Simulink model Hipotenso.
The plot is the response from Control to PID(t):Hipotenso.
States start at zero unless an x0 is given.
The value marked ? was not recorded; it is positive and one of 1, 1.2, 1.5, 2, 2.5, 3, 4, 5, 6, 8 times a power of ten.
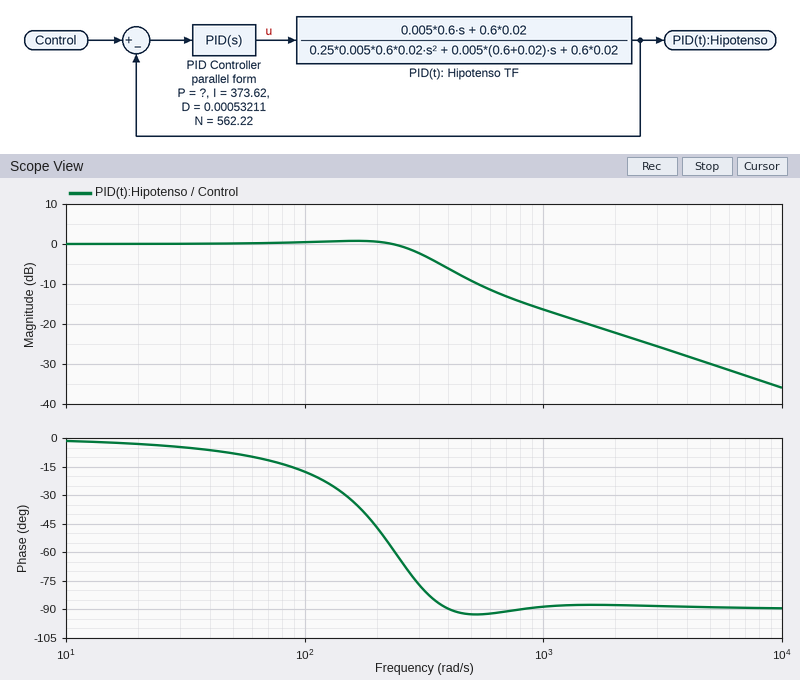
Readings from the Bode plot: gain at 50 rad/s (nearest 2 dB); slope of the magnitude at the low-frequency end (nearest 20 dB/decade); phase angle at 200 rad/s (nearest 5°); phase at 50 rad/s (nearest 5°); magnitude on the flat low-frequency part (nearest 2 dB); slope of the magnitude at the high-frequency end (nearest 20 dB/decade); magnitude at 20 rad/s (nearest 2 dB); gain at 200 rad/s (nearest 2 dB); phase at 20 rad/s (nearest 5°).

0 dB
0 dB/decade
-45°
-10°
0 dB
-20 dB/decade
0 dB
0 dB
-5°
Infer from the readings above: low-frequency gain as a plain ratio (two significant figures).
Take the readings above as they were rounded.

1.0
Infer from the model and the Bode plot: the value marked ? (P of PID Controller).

0.5
